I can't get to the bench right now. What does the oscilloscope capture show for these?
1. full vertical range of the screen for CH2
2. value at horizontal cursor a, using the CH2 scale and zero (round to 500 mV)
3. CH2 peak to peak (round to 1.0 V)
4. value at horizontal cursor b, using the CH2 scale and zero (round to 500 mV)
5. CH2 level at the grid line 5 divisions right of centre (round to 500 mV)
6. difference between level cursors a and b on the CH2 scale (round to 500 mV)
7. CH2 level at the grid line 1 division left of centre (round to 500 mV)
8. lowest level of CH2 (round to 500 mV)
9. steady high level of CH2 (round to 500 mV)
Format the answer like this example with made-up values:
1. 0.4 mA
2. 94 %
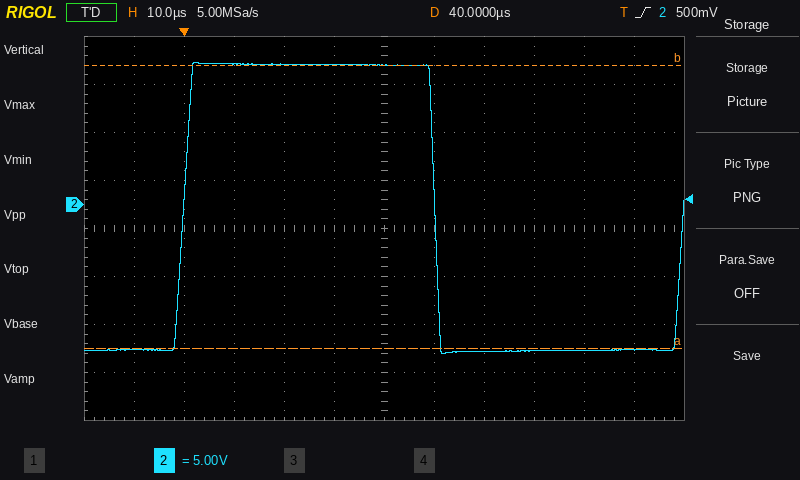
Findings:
1. 40 V
2. -15.0 V
3. 30.0 V
4. 14.5 V
5. -15.0 V
6. 29.5 V
7. 14.5 V
8. -15.5 V
9. 14.5 V
